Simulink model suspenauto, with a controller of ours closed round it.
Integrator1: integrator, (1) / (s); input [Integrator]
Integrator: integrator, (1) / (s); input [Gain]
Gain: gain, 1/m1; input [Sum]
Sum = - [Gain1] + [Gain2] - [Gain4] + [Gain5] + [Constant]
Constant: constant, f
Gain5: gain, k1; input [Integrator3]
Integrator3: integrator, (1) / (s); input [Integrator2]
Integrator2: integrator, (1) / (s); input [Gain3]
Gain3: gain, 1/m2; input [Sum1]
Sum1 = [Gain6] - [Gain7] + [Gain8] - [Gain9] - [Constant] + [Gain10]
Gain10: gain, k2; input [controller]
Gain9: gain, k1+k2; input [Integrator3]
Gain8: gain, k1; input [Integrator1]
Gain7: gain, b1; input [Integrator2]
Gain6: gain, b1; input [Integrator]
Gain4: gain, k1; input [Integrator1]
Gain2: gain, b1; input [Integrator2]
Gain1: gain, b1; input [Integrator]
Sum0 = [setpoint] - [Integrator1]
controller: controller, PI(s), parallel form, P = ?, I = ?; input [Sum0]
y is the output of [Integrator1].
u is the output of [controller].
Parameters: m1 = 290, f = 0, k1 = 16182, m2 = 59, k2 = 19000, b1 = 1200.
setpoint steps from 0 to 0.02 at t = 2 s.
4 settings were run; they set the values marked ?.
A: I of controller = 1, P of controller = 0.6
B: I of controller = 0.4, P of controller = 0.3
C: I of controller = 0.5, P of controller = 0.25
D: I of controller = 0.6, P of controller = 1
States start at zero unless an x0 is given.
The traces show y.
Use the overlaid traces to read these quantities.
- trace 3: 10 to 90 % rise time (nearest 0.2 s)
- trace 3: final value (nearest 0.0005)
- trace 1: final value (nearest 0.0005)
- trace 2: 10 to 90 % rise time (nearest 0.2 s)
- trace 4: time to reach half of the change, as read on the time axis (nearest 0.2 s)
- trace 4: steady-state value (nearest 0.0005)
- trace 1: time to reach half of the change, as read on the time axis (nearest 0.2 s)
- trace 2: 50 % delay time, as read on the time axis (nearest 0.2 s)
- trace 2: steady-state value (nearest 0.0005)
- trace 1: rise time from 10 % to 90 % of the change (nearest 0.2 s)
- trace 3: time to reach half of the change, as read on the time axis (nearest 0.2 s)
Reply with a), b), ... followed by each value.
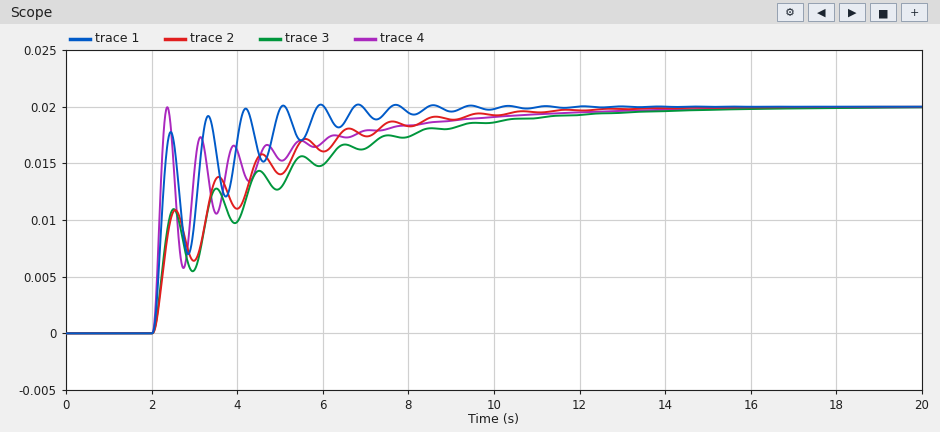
a) 6.2 s
b) 0.0200
c) 0.0200
d) 4.4 s
e) 2.2 s
f) 0.0200
g) 2.2 s
h) 2.4 s
i) 0.0200
j) 1.2 s
k) 2.4 s
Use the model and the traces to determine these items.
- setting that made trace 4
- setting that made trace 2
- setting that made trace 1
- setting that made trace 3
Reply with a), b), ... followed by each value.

a) D
b) C
c) A
d) B
